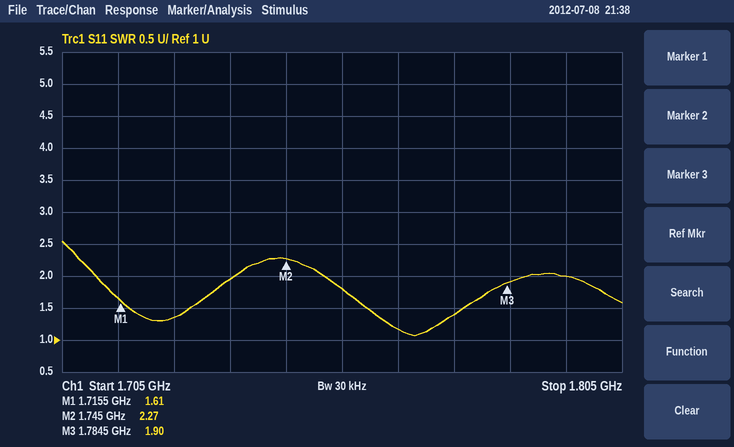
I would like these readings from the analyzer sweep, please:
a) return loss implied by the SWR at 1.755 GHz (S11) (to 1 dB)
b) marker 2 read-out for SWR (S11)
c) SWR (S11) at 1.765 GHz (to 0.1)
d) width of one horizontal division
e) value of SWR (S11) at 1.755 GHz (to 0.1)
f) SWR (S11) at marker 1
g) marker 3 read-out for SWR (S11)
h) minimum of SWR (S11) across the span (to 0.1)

11 dB
2.27
1.2
10 MHz
1.8
1.61
1.90
1.1
